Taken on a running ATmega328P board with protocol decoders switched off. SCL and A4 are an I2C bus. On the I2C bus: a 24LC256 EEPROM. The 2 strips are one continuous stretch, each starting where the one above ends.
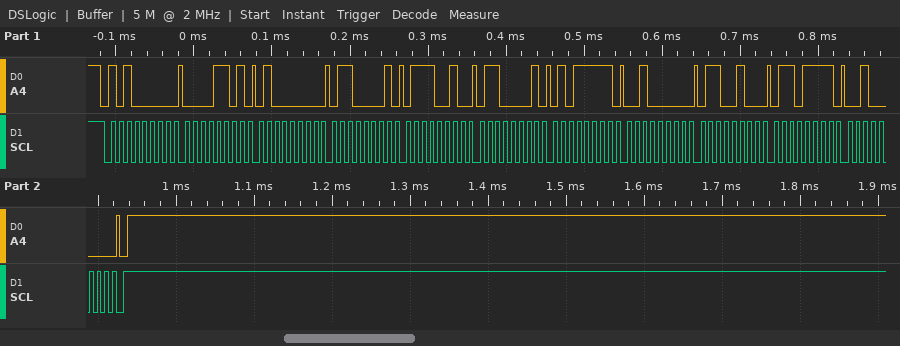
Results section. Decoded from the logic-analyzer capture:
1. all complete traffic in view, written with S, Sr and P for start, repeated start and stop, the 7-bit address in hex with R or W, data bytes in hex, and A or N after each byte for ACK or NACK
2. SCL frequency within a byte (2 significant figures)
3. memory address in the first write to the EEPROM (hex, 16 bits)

S 50W A 0D A 40 A 61 A 72 A 61 A 5F A 20 A 64 A 6F A 20 A P
100 kHz
0x0D40
